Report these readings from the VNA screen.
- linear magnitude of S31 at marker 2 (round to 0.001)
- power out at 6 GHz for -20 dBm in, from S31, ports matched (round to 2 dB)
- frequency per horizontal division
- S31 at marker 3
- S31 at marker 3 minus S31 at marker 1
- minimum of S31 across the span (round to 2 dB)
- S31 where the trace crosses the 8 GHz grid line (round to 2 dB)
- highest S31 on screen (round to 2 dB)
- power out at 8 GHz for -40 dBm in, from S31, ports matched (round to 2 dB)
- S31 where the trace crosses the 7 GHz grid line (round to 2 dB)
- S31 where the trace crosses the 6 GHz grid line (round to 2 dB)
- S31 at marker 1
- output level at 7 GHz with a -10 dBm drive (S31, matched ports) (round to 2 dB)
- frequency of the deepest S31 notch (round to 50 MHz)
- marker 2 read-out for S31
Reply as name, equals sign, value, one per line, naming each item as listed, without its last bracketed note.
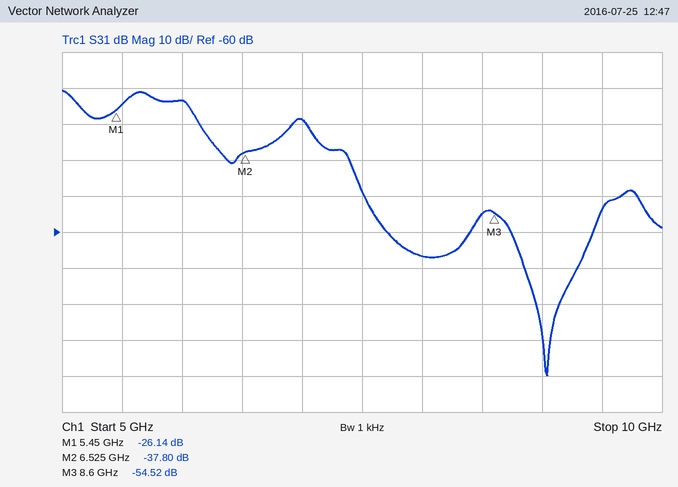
linear magnitude of S31 at marker 2 = 0.013
power out at 6 GHz for -20 dBm in, from S31, ports matched = -44 dBm
frequency per horizontal division = 500 MHz
S31 at marker 3 = -54.52 dB
S31 at marker 3 minus S31 at marker 1 = -28.38 dB
minimum of S31 across the span = -100 dB
S31 where the trace crosses the 8 GHz grid line = -66 dB
highest S31 on screen = -20 dB
power out at 8 GHz for -40 dBm in, from S31, ports matched = -106 dBm
S31 where the trace crosses the 7 GHz grid line = -28 dB
S31 where the trace crosses the 6 GHz grid line = -24 dB
S31 at marker 1 = -26.14 dB
output level at 7 GHz with a -10 dBm drive (S31, matched ports) = -38 dBm
frequency of the deepest S31 notch = 9.05 GHz
marker 2 read-out for S31 = -37.80 dB
